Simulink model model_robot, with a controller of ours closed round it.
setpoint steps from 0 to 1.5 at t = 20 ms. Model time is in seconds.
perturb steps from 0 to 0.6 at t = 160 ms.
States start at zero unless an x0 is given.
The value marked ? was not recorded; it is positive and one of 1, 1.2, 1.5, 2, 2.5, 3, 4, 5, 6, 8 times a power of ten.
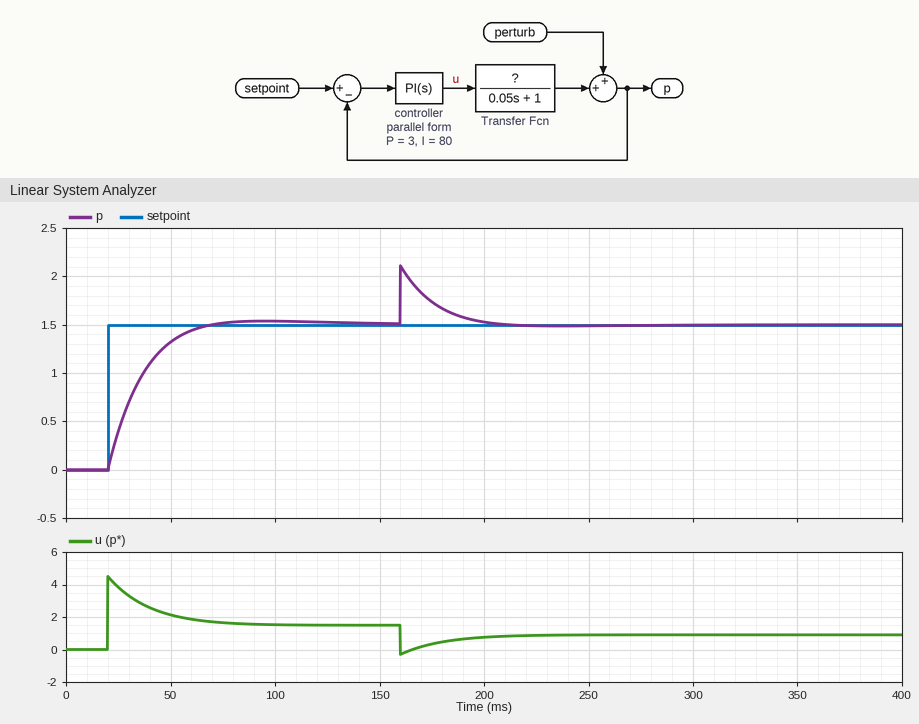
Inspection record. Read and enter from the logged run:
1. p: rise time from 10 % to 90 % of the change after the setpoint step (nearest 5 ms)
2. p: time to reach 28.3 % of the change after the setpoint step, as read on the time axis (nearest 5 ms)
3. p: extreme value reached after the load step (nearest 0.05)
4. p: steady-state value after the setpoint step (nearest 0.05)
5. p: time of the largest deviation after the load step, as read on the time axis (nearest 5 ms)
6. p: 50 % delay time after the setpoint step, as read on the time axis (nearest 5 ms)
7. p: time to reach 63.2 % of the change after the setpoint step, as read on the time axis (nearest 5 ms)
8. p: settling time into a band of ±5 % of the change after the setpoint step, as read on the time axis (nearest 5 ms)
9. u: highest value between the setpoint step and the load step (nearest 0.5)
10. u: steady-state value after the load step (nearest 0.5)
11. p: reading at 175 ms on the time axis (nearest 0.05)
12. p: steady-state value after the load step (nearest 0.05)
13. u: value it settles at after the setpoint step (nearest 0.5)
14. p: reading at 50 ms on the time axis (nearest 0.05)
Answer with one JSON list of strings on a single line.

["30 ms", "25 ms", "2.10", "1.50", "160 ms", "30 ms", "35 ms", "60 ms", "4.5", "1.0", "1.75", "1.50", "1.5", "1.30"]
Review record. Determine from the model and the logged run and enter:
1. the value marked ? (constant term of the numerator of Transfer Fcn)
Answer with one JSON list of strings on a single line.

["1"]
